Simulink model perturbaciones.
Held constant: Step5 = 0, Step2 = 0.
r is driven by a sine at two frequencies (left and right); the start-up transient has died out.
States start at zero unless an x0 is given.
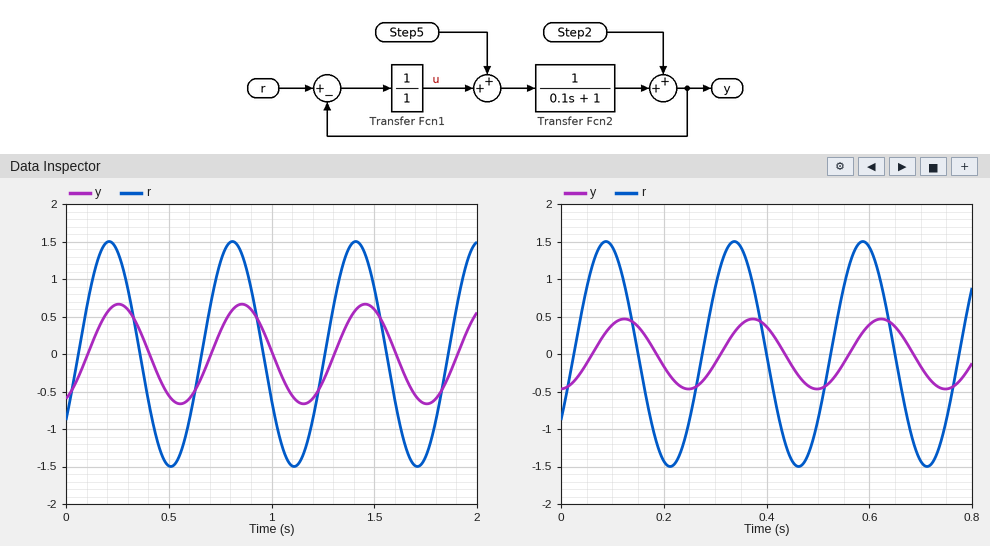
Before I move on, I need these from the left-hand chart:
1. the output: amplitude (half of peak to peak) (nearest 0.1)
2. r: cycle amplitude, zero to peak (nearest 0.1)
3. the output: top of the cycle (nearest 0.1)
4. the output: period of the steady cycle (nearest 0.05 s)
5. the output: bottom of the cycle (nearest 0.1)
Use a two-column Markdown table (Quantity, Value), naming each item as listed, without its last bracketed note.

| Quantity | Value |
|---|---|
| the output: amplitude (half of peak to peak) | 0.7 |
| r: cycle amplitude, zero to peak | 1.5 |
| the output: top of the cycle | 0.7 |
| the output: period of the steady cycle | 0.60 s |
| the output: bottom of the cycle | -0.7 |
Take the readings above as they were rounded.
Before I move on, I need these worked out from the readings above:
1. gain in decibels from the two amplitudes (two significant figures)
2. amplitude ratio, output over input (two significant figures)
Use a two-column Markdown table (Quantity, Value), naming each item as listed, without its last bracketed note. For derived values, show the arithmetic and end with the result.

| Quantity | Value |
|---|---|
| gain in decibels from the two amplitudes | 20 log10(0.7 / 1.5) = -6.6 dB |
| amplitude ratio, output over input | 0.7 / 1.5 = 0.47 |
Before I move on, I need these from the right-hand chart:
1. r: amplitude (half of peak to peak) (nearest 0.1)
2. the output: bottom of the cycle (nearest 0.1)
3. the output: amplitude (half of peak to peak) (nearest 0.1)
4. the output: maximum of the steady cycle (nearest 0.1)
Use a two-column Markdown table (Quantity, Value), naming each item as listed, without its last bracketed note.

| Quantity | Value |
|---|---|
| r: amplitude (half of peak to peak) | 1.5 |
| the output: bottom of the cycle | -0.5 |
| the output: amplitude (half of peak to peak) | 0.5 |
| the output: maximum of the steady cycle | 0.5 |
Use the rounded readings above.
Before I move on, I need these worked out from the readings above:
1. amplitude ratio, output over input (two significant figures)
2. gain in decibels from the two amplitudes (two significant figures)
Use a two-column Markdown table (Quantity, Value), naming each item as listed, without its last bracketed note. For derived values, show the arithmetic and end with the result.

| Quantity | Value |
|---|---|
| amplitude ratio, output over input | 0.5 / 1.5 = 0.33 |
| gain in decibels from the two amplitudes | 20 log10(0.5 / 1.5) = -9.5 dB |
